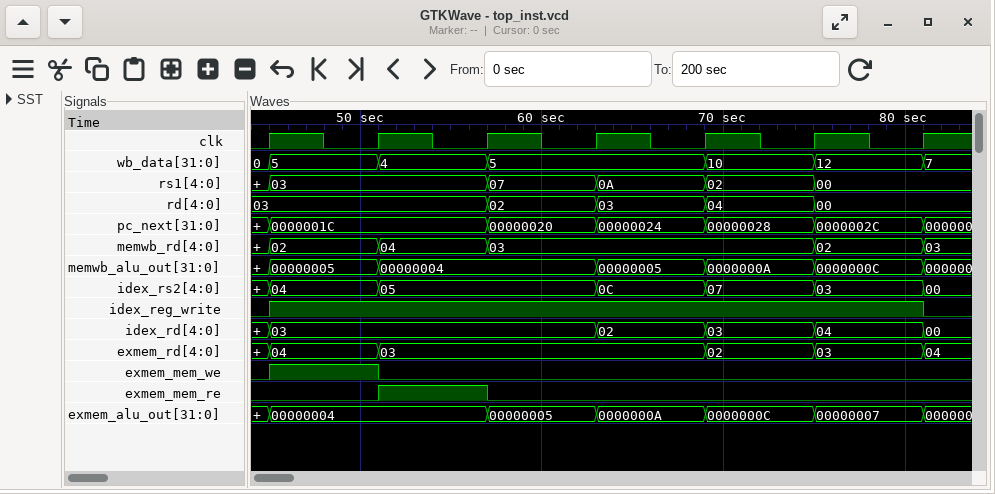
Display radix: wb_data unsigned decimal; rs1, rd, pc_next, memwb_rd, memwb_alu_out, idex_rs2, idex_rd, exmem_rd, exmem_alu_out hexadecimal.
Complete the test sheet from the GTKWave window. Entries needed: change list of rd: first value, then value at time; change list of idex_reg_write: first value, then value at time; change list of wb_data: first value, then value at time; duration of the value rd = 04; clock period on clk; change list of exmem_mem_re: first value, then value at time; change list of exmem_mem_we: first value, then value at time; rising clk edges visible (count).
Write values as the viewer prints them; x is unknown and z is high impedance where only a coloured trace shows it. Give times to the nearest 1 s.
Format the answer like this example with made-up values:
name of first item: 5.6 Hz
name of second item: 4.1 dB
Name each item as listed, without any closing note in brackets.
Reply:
change list of rd: first value, then value at time: 03, 02 at 57 s, 03 at 63 s, 04 at 69 s, 00 at 75 s
change list of idex_reg_write: first value, then value at time: 0, 1 at 45 s, 0 at 81 s
change list of wb_data: first value, then value at time: 0, 5 at 45 s, 4 at 51 s, 5 at 57 s, 10 at 69 s, 12 at 75 s, 7 at 81 s
duration of the value rd = 04: 6 s
clock period on clk: 6 s
change list of exmem_mem_re: first value, then value at time: 0, 1 at 51 s, 0 at 57 s
change list of exmem_mem_we: first value, then value at time: 0, 1 at 45 s, 0 at 51 s
rising clk edges visible: 7
